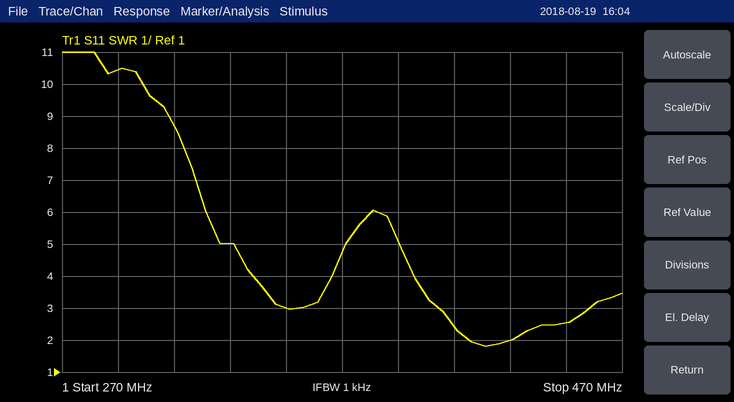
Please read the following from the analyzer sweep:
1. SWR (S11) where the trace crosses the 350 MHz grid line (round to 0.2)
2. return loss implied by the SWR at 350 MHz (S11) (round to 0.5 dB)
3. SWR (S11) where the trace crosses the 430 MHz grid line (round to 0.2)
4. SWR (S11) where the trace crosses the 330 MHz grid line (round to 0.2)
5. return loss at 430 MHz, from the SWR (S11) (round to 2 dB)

3.0
6.0 dB
2.0
5.0
10 dB
